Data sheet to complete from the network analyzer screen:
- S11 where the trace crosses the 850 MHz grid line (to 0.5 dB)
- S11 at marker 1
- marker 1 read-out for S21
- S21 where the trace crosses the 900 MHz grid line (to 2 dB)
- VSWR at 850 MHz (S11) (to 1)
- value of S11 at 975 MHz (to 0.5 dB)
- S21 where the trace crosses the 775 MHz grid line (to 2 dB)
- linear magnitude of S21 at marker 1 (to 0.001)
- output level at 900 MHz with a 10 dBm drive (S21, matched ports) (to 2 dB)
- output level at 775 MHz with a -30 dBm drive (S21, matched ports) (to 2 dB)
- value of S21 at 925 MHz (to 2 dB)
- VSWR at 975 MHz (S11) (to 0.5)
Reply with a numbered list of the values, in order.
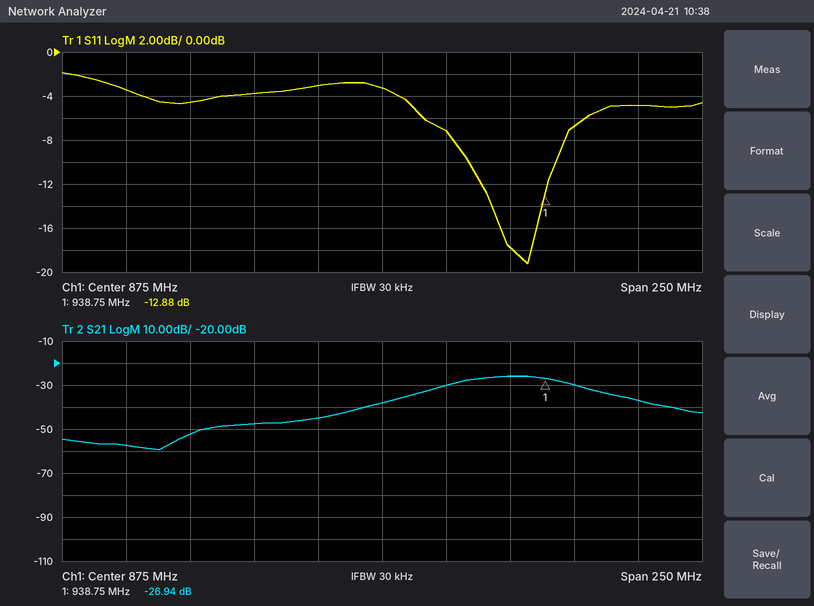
1. -3.0 dB
2. -12.88 dB
3. -26.94 dB
4. -30 dB
5. 6
6. -5.0 dB
7. -58 dB
8. 0.045
9. -20 dBm
10. -88 dBm
11. -26 dB
12. 3.5
